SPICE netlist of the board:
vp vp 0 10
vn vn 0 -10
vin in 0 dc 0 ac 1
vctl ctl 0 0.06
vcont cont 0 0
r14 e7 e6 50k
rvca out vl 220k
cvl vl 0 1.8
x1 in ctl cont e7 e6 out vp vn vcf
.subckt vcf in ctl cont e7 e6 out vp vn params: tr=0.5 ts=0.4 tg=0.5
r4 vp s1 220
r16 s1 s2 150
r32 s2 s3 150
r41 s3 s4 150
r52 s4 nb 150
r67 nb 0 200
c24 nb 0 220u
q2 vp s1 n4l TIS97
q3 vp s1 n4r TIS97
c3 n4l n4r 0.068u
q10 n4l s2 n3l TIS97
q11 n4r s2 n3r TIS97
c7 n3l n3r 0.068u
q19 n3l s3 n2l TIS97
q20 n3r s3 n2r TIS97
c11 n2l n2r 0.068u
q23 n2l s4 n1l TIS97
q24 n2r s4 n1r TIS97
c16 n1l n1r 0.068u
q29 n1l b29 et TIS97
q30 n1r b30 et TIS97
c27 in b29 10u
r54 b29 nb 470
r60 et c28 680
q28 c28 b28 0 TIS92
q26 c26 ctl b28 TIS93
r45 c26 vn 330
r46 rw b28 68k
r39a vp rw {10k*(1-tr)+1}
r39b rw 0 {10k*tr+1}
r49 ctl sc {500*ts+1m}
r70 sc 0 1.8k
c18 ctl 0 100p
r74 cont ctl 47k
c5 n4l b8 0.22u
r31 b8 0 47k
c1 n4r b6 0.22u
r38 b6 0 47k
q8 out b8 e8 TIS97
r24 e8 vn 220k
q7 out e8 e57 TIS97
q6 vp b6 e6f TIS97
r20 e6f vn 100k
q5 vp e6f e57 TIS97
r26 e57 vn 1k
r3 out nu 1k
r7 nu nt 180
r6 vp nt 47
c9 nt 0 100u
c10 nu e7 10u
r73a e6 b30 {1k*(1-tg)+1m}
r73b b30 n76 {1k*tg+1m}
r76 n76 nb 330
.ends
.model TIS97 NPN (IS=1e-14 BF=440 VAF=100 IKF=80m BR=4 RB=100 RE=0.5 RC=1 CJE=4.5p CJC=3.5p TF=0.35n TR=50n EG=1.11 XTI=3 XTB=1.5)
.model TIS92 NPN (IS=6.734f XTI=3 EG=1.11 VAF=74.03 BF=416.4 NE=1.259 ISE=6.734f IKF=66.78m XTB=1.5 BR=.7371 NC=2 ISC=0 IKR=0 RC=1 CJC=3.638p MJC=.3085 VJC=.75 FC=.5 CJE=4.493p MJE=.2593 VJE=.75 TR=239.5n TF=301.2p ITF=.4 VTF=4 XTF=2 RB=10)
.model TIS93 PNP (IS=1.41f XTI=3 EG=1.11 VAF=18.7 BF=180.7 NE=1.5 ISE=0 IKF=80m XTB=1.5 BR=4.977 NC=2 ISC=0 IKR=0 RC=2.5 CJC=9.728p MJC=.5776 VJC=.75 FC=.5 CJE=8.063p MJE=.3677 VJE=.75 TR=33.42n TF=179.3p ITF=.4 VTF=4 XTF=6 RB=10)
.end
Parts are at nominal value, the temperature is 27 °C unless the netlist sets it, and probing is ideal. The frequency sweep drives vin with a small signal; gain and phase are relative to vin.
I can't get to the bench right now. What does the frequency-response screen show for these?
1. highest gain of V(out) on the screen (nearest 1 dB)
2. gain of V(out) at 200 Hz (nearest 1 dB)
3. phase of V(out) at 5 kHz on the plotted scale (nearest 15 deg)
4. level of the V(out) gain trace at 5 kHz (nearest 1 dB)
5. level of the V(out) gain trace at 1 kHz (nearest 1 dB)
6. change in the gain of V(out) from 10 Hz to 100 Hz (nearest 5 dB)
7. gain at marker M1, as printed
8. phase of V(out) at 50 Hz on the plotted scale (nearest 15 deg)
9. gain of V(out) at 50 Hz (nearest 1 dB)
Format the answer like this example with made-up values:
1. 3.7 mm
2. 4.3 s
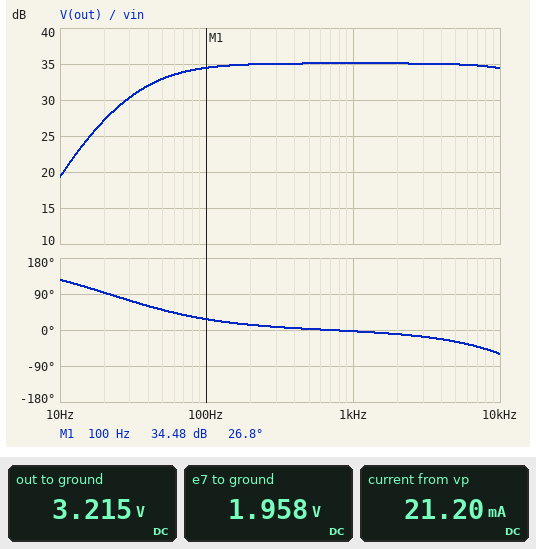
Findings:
1. 35 dB
2. 35 dB
3. -30 deg
4. 35 dB
5. 35 dB
6. 15 dB
7. 34.48 dB
8. 45 deg
9. 33 dB
